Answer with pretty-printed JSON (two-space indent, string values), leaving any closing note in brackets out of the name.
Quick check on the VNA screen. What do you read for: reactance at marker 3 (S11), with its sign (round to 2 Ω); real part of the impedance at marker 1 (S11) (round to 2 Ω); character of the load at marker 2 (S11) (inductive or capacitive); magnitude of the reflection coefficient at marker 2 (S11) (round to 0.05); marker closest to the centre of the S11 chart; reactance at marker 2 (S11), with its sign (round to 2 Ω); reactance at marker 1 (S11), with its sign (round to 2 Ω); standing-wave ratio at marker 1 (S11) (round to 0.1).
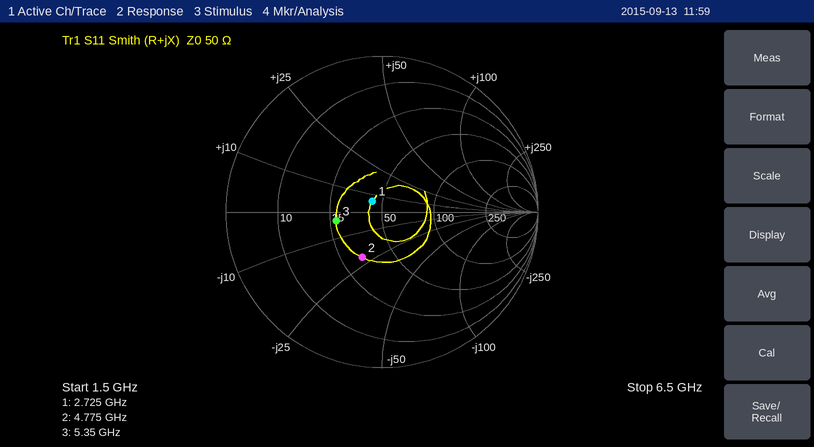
{
  "reactance at marker 3 (S11), with its sign": "-4 Ω",
  "real part of the impedance at marker 1 (S11)": "44 Ω",
  "character of the load at marker 2 (S11)": "capacitive",
  "magnitude of the reflection coefficient at marker 2 (S11)": "0.30",
  "marker closest to the centre of the S11 chart": "marker 1",
  "reactance at marker 2 (S11), with its sign": "-22 Ω",
  "reactance at marker 1 (S11), with its sign": "+6 Ω",
  "standing-wave ratio at marker 1 (S11)": "1.2"
}
